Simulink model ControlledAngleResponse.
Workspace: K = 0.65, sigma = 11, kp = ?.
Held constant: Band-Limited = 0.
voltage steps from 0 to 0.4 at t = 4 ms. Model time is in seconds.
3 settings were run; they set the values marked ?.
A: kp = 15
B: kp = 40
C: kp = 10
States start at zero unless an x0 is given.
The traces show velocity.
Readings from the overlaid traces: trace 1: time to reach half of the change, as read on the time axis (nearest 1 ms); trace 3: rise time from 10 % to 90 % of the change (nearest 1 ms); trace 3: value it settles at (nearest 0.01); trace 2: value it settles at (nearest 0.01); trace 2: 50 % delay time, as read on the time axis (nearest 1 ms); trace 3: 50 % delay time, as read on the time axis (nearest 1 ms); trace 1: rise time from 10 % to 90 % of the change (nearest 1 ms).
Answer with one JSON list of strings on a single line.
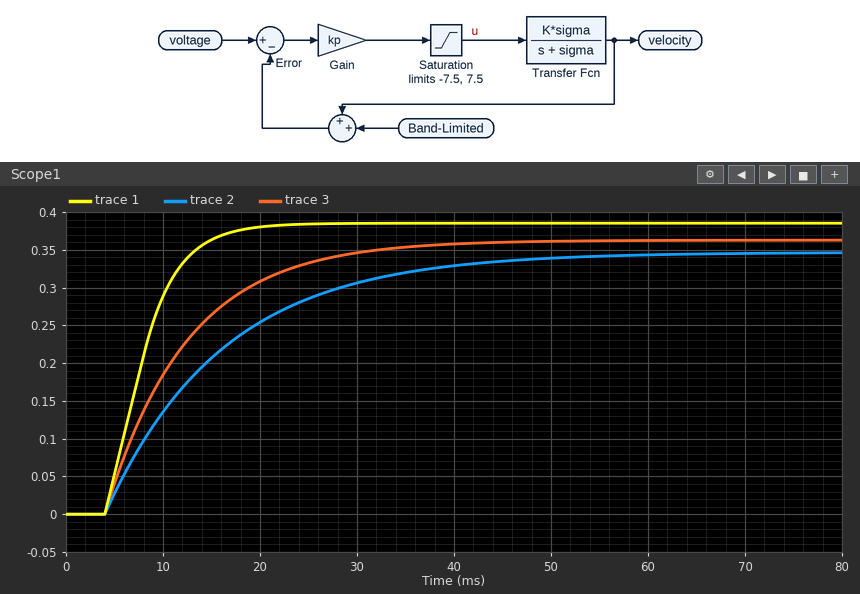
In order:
["8 ms", "19 ms", "0.36", "0.35", "12 ms", "10 ms", "8 ms"]
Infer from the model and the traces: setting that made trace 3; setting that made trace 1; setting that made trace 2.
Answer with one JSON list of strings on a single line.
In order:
["A", "B", "C"]
